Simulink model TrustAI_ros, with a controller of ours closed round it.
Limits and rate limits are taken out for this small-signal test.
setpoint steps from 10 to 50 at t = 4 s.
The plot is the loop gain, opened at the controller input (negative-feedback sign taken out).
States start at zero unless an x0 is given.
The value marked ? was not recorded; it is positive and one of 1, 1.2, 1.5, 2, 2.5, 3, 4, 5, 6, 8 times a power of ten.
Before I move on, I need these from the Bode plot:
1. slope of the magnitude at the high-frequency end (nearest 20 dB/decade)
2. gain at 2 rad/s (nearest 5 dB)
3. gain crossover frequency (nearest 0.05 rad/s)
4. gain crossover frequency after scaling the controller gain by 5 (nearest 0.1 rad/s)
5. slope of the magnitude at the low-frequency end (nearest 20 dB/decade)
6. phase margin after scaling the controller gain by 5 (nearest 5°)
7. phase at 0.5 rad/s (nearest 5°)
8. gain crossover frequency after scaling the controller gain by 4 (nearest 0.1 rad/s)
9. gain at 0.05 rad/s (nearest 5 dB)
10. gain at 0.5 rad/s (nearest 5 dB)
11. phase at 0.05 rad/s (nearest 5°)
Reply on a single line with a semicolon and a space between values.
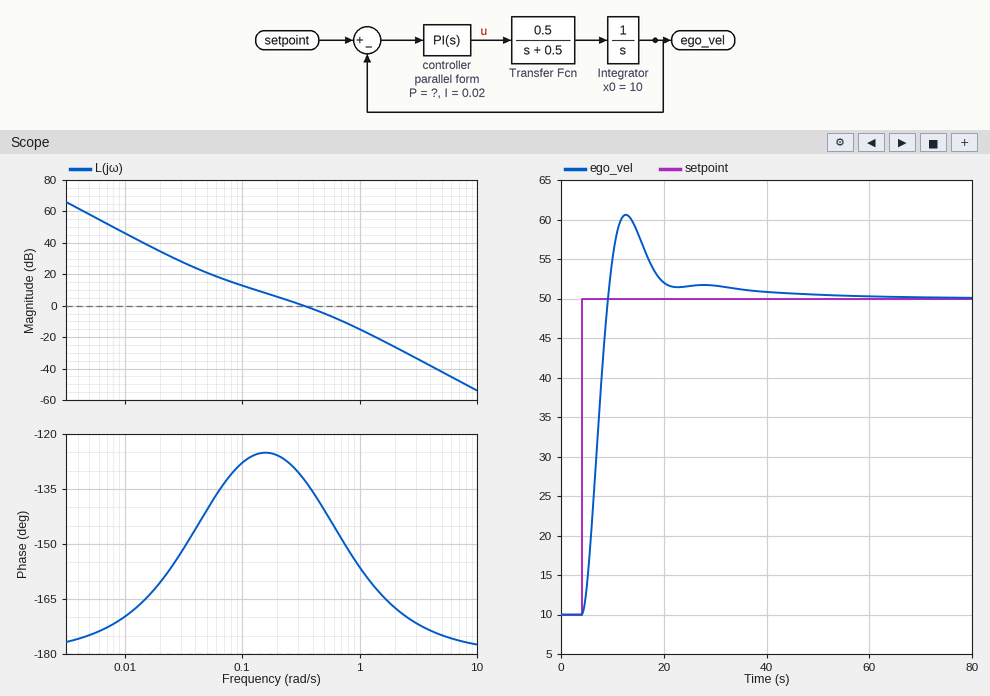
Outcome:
-40 dB/decade; -25 dB; 0.35 rad/s; 0.9 rad/s; -40 dB/decade; 25°; -140°; 0.8 rad/s; 20 dB; -5 dB; -140°
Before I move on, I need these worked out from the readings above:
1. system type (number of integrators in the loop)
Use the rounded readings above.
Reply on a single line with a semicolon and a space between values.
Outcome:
2
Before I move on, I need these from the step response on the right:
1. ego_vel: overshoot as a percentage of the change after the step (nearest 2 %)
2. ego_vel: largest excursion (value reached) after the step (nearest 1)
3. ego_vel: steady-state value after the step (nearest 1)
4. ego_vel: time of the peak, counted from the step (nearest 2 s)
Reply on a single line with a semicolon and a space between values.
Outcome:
26 %; 61; 50; 8 s
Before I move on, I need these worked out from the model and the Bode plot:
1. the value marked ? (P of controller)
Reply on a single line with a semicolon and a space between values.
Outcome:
0.4
